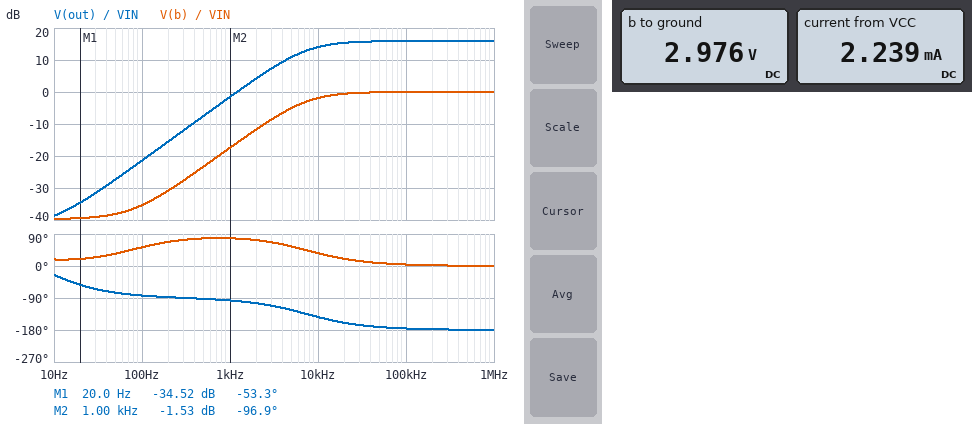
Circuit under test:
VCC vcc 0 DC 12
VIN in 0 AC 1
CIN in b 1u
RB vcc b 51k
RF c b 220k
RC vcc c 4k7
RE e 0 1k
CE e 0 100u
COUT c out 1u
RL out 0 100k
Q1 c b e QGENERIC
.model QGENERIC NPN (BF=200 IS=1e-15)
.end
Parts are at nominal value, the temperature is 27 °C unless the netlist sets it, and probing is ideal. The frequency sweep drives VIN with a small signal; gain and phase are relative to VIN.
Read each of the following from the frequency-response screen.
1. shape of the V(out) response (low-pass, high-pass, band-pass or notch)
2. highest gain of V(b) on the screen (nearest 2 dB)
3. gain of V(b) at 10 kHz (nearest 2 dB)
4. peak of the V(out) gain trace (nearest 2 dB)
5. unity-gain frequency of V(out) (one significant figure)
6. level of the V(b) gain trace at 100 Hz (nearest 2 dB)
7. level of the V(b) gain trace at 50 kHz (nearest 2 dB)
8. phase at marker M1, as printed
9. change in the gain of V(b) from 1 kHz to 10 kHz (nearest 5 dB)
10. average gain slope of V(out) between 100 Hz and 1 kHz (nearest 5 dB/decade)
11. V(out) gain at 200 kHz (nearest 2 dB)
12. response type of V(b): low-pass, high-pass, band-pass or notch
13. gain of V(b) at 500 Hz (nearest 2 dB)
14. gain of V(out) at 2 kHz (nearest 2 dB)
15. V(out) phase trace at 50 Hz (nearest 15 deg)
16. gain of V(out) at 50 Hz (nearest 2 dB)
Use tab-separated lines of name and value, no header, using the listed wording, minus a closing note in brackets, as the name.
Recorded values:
shape of the V(out) response	high-pass
highest gain of V(b) on the screen	0 dB
gain of V(b) at 10 kHz	-2 dB
peak of the V(out) gain trace	16 dB
unity-gain frequency of V(out)	1 kHz
level of the V(b) gain trace at 100 Hz	-36 dB
level of the V(b) gain trace at 50 kHz	0 dB
phase at marker M1, as printed	-53.3 deg
change in the gain of V(b) from 1 kHz to 10 kHz	15 dB
average gain slope of V(out) between 100 Hz and 1 kHz	20 dB/decade
V(out) gain at 200 kHz	16 dB
response type of V(b): low-pass, high-pass, band-pass or notch	high-pass
gain of V(b) at 500 Hz	-24 dB
gain of V(out) at 2 kHz	4 dB
V(out) phase trace at 50 Hz	-75 deg
gain of V(out) at 50 Hz	-28 dB
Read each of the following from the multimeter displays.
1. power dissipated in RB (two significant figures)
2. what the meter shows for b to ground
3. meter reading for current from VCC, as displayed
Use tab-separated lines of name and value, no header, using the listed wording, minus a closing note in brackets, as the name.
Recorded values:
power dissipated in RB	1.6 mW
what the meter shows for b to ground	2.976 V
meter reading for current from VCC, as displayed	2.239 mA
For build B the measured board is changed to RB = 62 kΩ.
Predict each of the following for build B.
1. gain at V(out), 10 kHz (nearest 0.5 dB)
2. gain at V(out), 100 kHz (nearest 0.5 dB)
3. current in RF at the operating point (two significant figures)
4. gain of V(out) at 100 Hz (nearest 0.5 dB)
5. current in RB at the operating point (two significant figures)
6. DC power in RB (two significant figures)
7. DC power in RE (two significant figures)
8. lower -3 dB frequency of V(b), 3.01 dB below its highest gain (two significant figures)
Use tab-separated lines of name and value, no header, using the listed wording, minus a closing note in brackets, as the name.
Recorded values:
gain at V(out), 10 kHz	16.0 dB
gain at V(out), 100 kHz	17.5 dB
current in RF at the operating point	3.0 µA
gain of V(out) at 100 Hz	-19.5 dB
current in RB at the operating point	150 µA
DC power in RB	1.3 mW
DC power in RE	4.9 mW
lower -3 dB frequency of V(b), 3.01 dB below its highest gain	7.2 kHz
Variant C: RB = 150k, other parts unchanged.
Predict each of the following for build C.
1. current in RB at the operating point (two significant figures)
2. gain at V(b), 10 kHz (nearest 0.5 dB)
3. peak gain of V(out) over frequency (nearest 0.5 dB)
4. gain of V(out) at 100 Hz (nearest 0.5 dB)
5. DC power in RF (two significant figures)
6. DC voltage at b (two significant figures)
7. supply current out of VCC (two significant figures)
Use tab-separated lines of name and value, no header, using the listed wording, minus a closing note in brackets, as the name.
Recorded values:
current in RB at the operating point	61 µA
gain at V(b), 10 kHz	-1.5 dB
peak gain of V(out) over frequency	26.5 dB
gain of V(out) at 100 Hz	-10.0 dB
DC power in RF	1.8 µW
DC voltage at b	2.9 V
supply current out of VCC	2.1 mA
